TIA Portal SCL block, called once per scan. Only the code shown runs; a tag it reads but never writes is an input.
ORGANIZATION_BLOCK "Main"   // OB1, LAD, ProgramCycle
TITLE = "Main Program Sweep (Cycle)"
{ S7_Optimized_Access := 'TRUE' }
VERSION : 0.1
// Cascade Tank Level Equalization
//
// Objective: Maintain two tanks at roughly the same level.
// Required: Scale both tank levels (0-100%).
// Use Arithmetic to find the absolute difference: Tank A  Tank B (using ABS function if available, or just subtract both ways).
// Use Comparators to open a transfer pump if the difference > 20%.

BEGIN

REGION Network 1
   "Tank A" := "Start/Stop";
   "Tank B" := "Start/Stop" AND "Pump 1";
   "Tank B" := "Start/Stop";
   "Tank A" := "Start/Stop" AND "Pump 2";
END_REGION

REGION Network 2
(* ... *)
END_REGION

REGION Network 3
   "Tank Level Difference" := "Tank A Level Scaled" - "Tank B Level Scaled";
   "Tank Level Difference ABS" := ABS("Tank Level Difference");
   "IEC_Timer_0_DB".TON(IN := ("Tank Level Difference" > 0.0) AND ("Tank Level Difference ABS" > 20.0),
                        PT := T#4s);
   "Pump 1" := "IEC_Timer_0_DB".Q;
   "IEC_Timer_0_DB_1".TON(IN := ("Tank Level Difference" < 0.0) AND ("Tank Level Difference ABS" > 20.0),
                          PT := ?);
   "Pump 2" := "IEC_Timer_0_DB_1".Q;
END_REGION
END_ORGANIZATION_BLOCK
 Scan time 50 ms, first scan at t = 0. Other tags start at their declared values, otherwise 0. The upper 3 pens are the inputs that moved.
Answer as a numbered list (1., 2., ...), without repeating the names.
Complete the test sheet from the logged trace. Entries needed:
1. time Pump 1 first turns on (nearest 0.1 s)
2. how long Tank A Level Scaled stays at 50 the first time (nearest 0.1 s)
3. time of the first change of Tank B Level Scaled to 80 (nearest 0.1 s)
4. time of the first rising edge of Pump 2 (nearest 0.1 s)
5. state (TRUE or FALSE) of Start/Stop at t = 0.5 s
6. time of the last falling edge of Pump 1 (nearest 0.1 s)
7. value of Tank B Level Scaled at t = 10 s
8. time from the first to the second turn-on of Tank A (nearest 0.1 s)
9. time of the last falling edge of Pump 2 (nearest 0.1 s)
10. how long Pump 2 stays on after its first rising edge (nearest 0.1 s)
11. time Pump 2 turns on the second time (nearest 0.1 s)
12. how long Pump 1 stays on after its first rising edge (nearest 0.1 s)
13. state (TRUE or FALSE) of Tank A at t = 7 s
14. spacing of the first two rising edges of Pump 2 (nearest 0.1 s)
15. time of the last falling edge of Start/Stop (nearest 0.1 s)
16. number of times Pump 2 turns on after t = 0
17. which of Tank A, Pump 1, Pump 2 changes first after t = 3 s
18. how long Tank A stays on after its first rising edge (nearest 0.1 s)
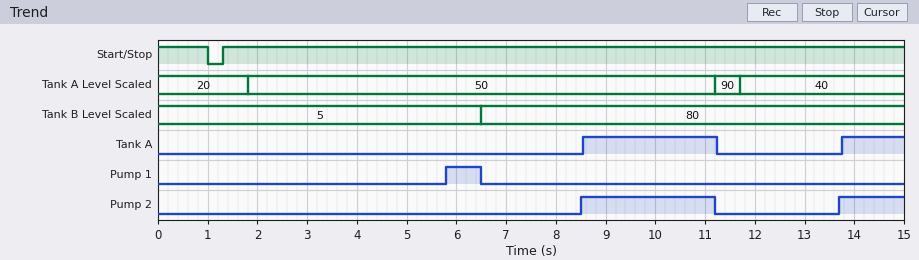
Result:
1. 5.8 s
2. 9.4 s
3. 6.5 s
4. 8.5 s
5. TRUE
6. 6.5 s
7. 80
8. 5.2 s
9. 11.2 s
10. 2.7 s
11. 13.7 s
12. 0.7 s
13. FALSE
14. 5.2 s
15. 1.0 s
16. 2
17. Pump 1
18. 2.7 s
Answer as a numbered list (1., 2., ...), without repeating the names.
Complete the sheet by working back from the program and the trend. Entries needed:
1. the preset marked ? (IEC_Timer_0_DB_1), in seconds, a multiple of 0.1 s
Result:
1. 2.0 s
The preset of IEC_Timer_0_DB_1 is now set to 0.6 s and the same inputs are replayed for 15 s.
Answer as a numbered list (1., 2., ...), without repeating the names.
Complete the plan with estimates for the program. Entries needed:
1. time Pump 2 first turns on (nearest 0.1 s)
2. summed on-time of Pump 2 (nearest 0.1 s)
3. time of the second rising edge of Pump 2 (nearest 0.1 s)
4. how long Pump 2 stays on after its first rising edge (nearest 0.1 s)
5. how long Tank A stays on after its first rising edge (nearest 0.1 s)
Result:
1. 7.1 s
2. 6.8 s
3. 12.3 s
4. 4.1 s
5. 4.1 s
